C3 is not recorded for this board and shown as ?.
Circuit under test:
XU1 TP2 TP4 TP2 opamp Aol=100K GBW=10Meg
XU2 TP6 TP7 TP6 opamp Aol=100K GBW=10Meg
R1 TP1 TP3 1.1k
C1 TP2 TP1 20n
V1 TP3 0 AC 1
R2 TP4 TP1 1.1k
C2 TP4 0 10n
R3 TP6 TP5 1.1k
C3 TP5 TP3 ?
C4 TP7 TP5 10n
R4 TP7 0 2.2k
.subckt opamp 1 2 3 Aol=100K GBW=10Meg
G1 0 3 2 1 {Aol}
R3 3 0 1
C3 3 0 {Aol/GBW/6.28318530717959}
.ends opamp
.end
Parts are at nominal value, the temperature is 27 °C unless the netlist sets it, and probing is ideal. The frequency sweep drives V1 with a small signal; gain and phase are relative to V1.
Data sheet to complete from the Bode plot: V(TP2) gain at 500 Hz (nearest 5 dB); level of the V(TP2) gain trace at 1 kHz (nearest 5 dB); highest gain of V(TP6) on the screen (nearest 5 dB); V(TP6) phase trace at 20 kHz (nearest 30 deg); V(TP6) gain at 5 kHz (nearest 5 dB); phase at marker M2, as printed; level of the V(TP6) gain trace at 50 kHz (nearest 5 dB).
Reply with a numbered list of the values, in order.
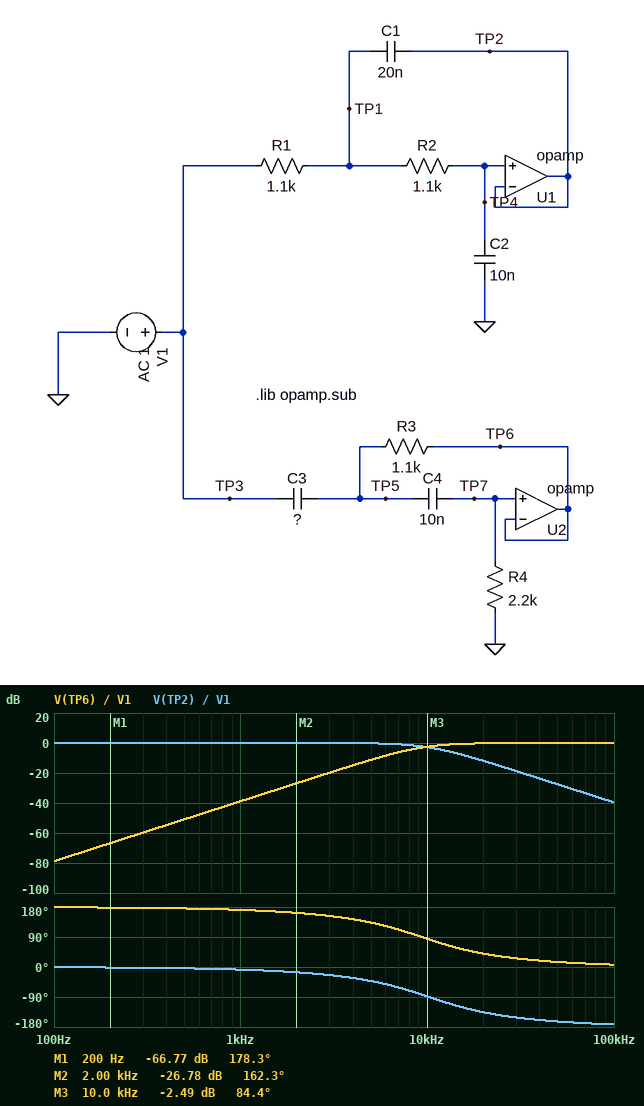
1. 0 dB
2. 0 dB
3. 0 dB
4. 30 deg
5. -10 dB
6. 162.3 deg
7. 0 dB
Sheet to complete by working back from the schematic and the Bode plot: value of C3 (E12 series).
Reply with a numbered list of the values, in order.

1. 12 nF
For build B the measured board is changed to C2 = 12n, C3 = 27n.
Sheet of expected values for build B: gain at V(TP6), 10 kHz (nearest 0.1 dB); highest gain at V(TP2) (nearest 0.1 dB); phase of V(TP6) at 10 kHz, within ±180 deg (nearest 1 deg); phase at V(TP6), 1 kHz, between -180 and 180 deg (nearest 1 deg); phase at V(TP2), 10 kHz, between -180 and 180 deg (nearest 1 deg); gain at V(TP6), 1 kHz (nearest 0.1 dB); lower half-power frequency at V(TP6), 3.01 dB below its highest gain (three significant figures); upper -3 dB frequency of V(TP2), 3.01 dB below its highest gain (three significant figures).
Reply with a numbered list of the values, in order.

1. -1.3 dB
2. 0 dB
3. 58 deg
4. 165 deg
5. -95 deg
6. -31.8 dB
7. 7.10 kHz
8. 8.46 kHz
